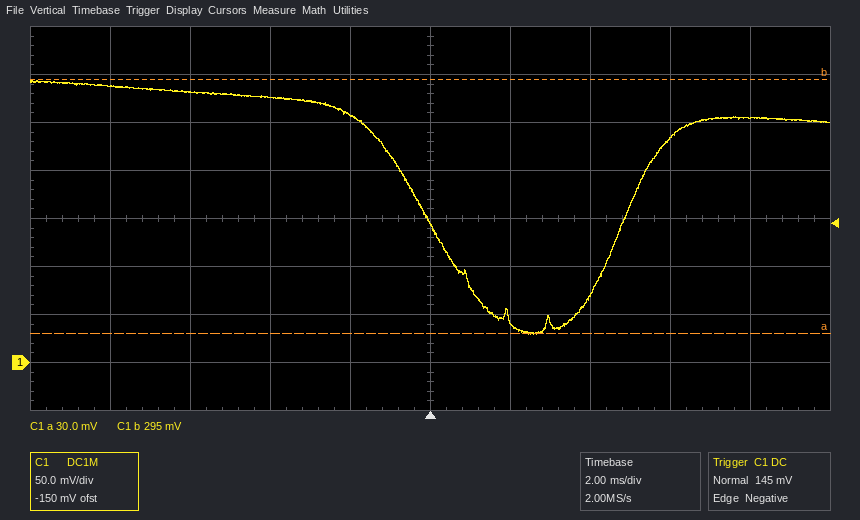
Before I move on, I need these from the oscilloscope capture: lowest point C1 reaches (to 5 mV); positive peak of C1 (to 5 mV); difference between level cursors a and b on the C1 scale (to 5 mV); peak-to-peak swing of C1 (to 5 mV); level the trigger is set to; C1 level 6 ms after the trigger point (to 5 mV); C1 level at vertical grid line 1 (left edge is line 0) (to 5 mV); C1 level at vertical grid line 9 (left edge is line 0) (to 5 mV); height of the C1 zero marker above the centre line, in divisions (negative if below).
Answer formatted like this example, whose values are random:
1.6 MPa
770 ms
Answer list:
30 mV
295 mV
265 mV
265 mV
145 mV
235 mV
290 mV
255 mV
-3.0 div
